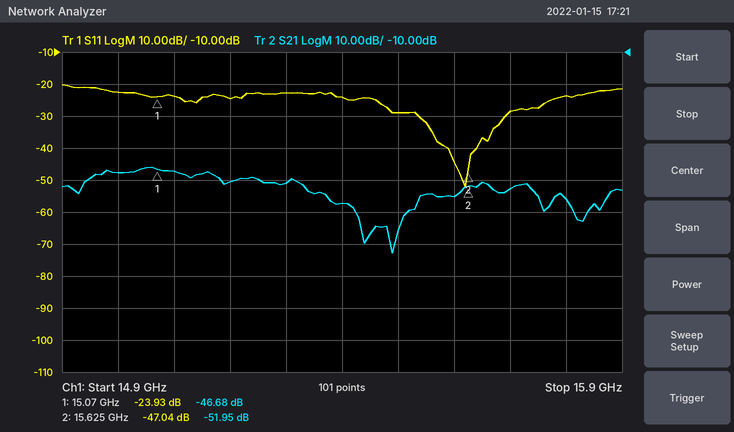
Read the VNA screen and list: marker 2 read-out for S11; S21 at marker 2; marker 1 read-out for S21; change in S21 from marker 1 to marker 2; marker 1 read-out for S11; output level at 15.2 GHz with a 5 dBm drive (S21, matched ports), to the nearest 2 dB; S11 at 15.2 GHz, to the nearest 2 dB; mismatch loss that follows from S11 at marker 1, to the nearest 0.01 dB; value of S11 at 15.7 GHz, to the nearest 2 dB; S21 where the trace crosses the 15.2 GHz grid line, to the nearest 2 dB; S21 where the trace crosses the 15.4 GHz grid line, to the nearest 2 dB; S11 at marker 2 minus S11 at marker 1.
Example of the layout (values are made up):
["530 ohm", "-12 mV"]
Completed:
["-47.04 dB", "-51.95 dB", "-46.68 dB", "-5.27 dB", "-23.93 dB", "-46 dBm", "-24 dB", "0.02 dB", "-28 dB", "-50 dB", "-58 dB", "-23.11 dB"]
